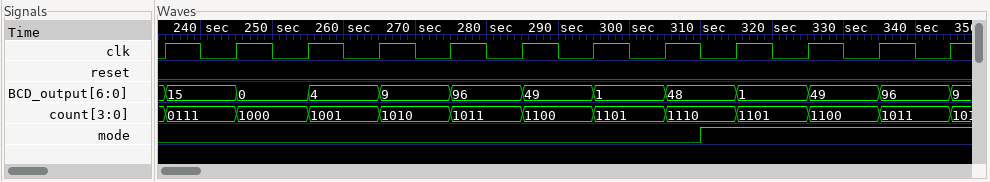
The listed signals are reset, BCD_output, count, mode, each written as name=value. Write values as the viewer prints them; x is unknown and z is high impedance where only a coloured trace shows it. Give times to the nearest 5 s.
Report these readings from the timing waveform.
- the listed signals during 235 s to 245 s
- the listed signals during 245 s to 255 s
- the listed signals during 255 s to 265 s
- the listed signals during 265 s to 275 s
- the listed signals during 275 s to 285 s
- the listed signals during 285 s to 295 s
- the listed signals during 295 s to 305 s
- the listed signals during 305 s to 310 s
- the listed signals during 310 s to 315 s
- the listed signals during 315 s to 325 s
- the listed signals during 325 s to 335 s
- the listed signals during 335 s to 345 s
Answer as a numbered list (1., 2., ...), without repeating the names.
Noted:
1. reset=0, BCD_output=15, count=0111, mode=0
2. reset=0, BCD_output=0, count=1000, mode=0
3. reset=0, BCD_output=4, count=1001, mode=0
4. reset=0, BCD_output=9, count=1010, mode=0
5. reset=0, BCD_output=96, count=1011, mode=0
6. reset=0, BCD_output=49, count=1100, mode=0
7. reset=0, BCD_output=1, count=1101, mode=0
8. reset=0, BCD_output=48, count=1110, mode=0
9. reset=0, BCD_output=48, count=1110, mode=1
10. reset=0, BCD_output=1, count=1101, mode=1
11. reset=0, BCD_output=49, count=1100, mode=1
12. reset=0, BCD_output=96, count=1011, mode=1
